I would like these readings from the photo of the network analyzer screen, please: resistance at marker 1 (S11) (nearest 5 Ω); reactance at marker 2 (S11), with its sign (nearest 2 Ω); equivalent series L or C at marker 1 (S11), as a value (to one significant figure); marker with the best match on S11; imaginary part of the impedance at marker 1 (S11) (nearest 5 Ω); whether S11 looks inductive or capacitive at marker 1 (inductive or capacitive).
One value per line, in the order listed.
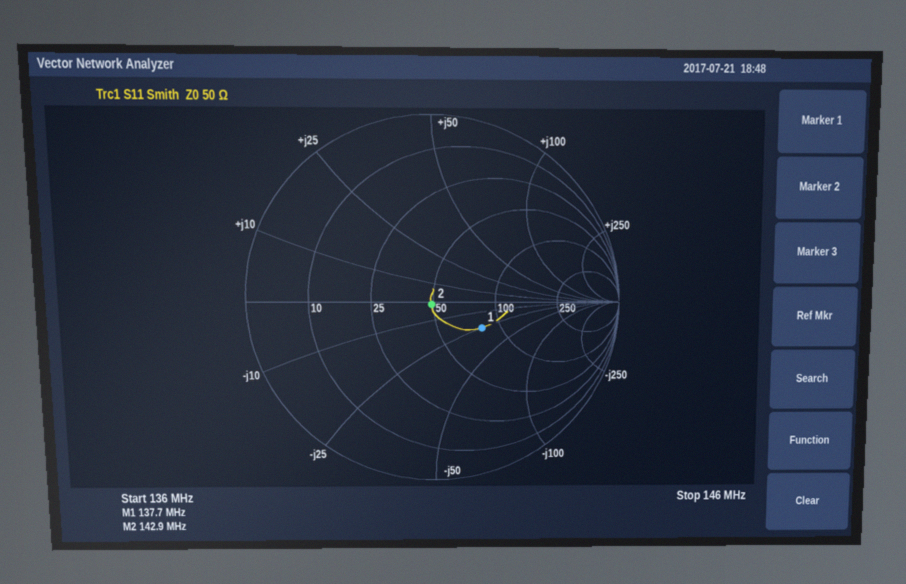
80 Ω
-2 Ω
50 pF
marker 2
-25 Ω
capacitive
